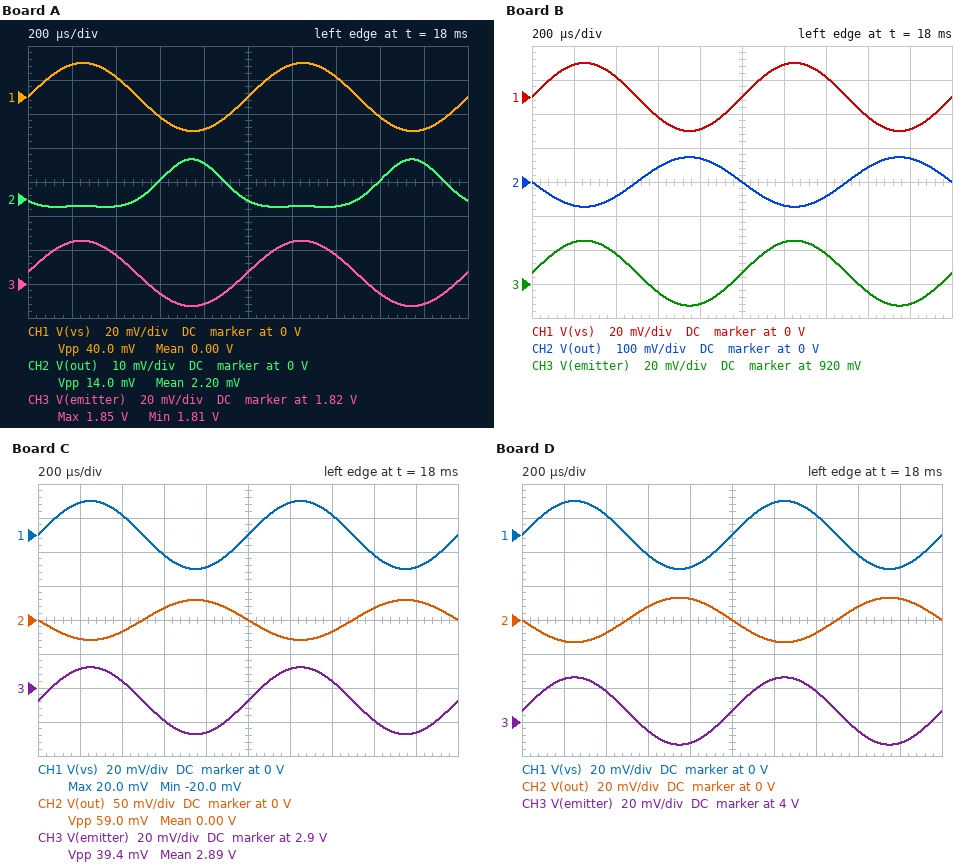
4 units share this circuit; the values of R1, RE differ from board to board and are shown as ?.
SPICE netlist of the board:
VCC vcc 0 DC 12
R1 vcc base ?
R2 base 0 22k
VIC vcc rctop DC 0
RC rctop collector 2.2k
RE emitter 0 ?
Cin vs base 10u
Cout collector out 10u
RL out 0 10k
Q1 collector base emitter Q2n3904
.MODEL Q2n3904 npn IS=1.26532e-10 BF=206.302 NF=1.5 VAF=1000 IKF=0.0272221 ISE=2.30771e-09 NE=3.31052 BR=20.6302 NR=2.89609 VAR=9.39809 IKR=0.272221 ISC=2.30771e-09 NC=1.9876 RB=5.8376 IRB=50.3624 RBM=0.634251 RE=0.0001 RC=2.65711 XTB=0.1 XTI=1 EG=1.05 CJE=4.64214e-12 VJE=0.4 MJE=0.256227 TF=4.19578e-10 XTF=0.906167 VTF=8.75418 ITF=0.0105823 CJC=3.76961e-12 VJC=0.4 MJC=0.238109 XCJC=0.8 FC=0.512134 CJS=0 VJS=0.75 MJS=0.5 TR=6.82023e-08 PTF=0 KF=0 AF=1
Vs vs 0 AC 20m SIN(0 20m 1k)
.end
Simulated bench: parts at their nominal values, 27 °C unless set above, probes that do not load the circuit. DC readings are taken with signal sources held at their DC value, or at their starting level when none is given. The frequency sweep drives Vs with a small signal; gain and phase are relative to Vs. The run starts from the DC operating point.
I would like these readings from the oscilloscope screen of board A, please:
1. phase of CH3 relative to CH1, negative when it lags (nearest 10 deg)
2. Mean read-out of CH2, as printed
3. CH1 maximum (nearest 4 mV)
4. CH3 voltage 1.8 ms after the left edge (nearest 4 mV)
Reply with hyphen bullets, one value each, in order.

- 0 deg
- 2.20 mV
- 20 mV
- 1.808 V
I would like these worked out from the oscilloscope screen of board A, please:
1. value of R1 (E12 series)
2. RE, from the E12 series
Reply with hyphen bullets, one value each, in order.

- 39 kΩ
- 390 Ω
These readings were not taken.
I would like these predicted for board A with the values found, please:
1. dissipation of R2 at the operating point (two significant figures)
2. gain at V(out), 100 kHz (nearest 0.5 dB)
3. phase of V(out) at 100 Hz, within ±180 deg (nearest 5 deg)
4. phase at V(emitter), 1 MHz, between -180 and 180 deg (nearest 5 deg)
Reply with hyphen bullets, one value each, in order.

- 290 µW
- -11.0 dB
- -160 deg
- 0 deg
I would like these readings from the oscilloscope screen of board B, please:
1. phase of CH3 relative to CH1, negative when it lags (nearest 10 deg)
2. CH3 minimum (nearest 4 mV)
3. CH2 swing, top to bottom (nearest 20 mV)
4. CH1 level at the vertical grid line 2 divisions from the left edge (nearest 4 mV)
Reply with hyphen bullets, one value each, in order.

- 0 deg
- 908 mV
- 140 mV
- 12 mV
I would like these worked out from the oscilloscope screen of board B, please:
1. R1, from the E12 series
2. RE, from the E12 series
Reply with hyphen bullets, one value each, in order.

- 120 kΩ
- 470 Ω
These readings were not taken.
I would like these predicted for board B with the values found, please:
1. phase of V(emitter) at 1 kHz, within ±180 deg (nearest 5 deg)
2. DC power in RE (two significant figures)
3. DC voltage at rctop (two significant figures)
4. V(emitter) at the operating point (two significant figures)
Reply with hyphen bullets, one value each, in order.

- 0 deg
- 1.8 mW
- 12 V
- 930 mV
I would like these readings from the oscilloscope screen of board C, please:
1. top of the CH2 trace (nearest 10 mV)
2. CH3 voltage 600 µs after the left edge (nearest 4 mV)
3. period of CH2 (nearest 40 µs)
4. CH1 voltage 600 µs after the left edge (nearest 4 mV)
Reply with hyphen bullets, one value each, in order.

- 30 mV
- 2.880 V
- 1.00 ms
- -12 mV
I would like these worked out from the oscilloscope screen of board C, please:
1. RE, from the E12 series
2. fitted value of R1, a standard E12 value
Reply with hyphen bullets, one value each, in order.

- 1.2 kΩ
- 47 kΩ
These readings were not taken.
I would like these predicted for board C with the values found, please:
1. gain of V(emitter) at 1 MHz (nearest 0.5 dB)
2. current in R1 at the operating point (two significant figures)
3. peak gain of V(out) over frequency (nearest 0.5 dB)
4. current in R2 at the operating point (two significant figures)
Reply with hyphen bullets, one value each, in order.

- 0 dB
- 180 µA
- 3.5 dB
- 160 µA
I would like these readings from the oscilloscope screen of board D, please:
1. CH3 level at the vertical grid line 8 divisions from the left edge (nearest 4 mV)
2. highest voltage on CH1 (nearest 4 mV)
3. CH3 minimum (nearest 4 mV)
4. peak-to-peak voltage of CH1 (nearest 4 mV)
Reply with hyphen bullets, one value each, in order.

- 3.996 V
- 20 mV
- 3.988 V
- 40 mV
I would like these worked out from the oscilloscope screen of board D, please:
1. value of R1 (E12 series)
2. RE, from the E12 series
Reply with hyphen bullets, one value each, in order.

- 33 kΩ
- 2.7 kΩ
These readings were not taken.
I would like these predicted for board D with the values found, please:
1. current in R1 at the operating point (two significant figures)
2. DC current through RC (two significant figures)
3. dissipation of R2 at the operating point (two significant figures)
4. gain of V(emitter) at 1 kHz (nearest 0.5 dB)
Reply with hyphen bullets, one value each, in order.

- 220 µA
- 1.5 mA
- 980 µW
- 0 dB
